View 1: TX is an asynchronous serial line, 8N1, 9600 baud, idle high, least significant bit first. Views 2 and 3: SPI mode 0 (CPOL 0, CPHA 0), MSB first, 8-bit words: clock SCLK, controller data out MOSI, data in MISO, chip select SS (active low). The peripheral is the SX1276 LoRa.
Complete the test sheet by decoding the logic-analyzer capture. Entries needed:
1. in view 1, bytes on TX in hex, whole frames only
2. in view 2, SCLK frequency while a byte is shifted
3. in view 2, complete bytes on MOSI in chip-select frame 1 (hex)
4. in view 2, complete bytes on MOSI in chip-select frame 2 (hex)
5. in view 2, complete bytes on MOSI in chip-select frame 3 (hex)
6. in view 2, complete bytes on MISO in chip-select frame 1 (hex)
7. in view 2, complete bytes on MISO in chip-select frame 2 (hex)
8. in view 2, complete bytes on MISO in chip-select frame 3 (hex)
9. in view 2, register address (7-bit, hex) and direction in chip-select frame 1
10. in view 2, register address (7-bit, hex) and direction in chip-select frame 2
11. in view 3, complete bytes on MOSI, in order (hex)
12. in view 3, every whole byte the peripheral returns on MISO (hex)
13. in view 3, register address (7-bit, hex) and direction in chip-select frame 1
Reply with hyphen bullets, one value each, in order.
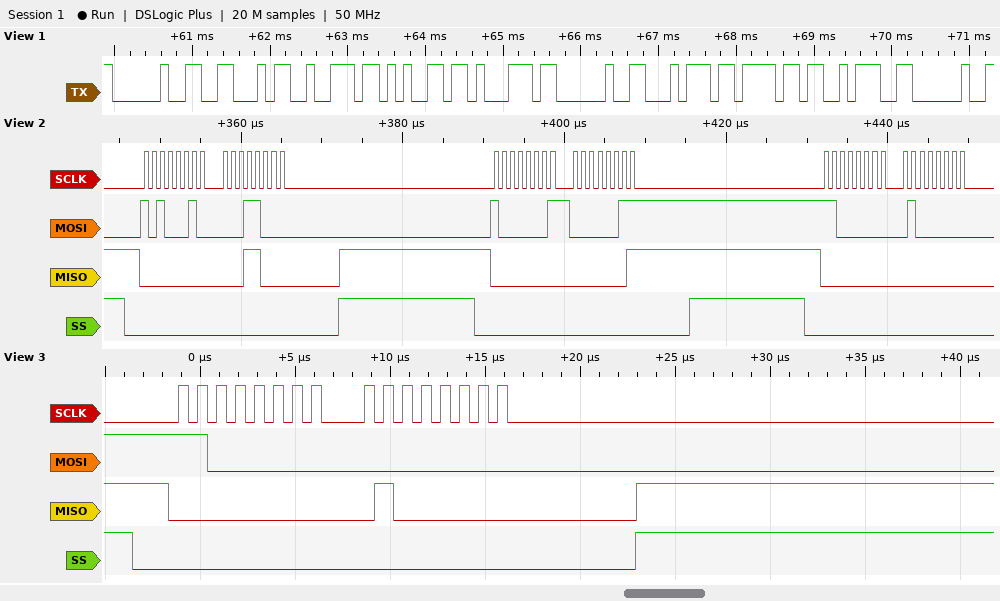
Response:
- 20 46 72 65 71 20 74 6F 3A 20
- 1 MHz
- 0xA2 0x18
- 0x81 0x03
- 0xC0 0x40
- 0x00 0x18
- 0x00 0x01
- 0x00 0x00
- 0x22 write
- 0x01 write
- C0 00
- 00 40
- 0x40 write
